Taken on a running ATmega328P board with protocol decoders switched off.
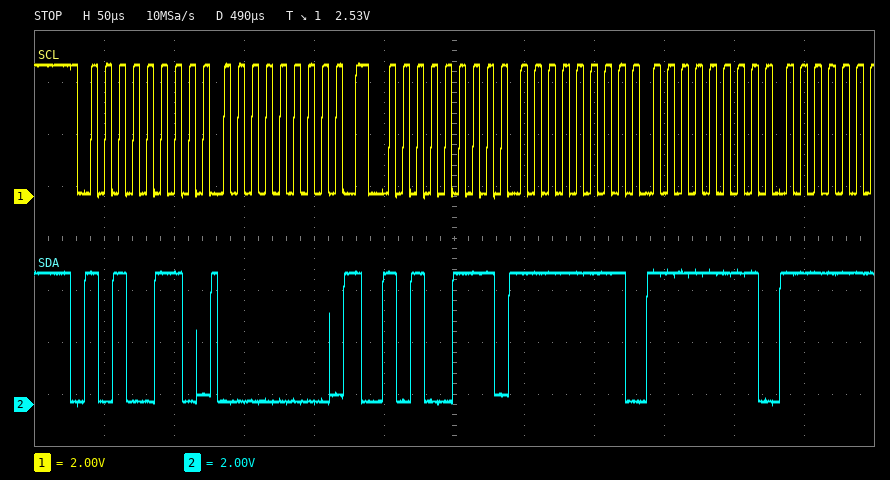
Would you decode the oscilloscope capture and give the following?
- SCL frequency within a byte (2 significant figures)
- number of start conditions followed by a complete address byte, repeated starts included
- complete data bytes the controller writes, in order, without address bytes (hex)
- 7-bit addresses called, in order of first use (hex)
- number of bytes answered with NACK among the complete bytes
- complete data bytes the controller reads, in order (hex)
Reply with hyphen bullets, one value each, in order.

- 100 kHz
- 2
- 00
- 0x53
- 0
- FF FF
